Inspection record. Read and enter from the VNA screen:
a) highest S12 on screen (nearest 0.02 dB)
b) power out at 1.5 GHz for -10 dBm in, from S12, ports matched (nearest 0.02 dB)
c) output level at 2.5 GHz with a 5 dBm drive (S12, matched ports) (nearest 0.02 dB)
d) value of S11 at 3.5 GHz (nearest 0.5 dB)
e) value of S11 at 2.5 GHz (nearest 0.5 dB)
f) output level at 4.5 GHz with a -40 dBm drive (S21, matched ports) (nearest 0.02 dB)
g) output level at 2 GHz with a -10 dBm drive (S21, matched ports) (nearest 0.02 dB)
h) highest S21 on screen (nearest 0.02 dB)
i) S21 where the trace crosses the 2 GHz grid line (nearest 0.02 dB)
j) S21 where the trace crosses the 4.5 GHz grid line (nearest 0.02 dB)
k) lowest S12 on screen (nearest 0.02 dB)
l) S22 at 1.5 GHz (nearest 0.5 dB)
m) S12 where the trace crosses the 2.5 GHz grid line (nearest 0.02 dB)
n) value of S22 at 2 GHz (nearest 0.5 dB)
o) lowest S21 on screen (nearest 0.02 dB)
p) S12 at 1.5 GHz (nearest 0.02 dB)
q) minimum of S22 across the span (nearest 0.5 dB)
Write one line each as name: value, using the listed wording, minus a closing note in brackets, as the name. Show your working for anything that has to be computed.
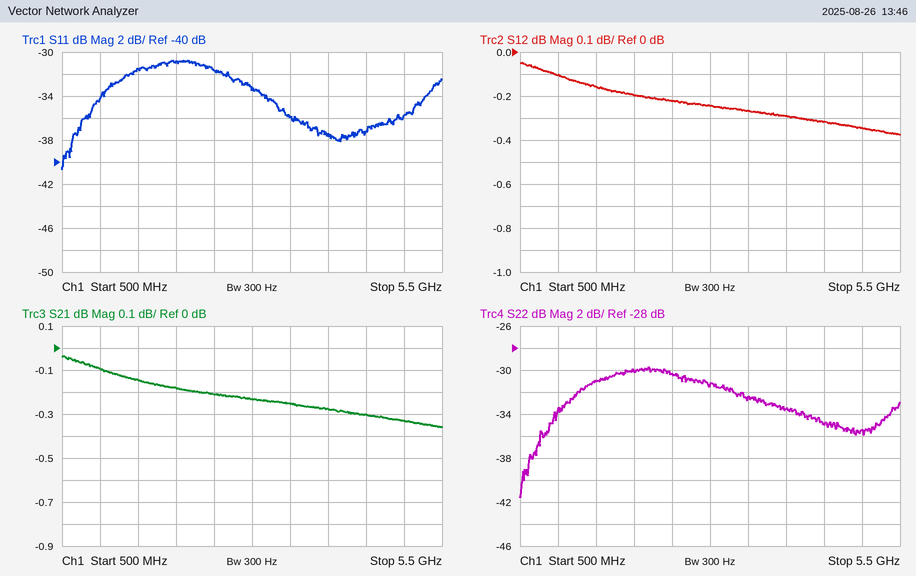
highest S12 on screen: -0.04 dB
power out at 1.5 GHz for -10 dBm in, from S12, ports matched: -10 dBm + (-0.16 dB) = -10.16 dBm
output level at 2.5 GHz with a 5 dBm drive (S12, matched ports): 5 dBm + (-0.22 dB) = 4.78 dBm
value of S11 at 3.5 GHz: -36.0 dB
value of S11 at 2.5 GHz: -31.5 dB
output level at 4.5 GHz with a -40 dBm drive (S21, matched ports): -40 dBm + (-0.30 dB) = -40.30 dBm
output level at 2 GHz with a -10 dBm drive (S21, matched ports): -10 dBm + (-0.18 dB) = -10.18 dBm
highest S21 on screen: -0.04 dB
S21 where the trace crosses the 2 GHz grid line: -0.18 dB
S21 where the trace crosses the 4.5 GHz grid line: -0.30 dB
lowest S12 on screen: -0.38 dB
S22 at 1.5 GHz: -31.0 dB
S12 where the trace crosses the 2.5 GHz grid line: -0.22 dB
value of S22 at 2 GHz: -30.0 dB
lowest S21 on screen: -0.36 dB
S12 at 1.5 GHz: -0.16 dB
minimum of S22 across the span: -41.5 dB
